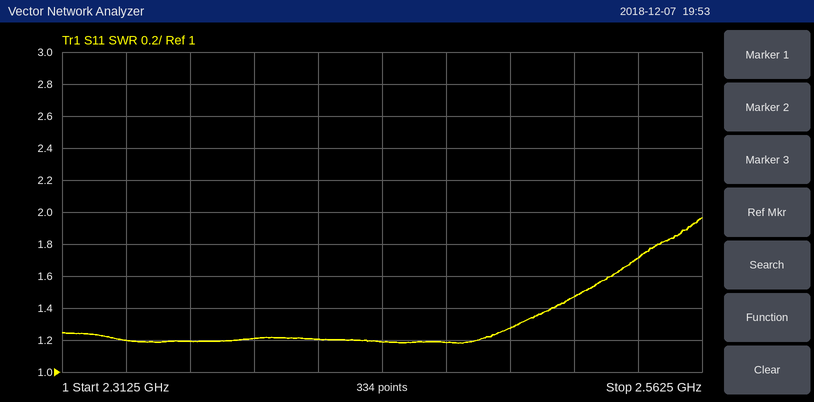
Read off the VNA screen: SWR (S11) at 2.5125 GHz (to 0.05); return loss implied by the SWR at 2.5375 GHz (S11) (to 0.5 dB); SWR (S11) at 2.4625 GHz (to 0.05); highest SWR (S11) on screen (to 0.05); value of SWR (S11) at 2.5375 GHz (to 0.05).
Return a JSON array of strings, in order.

["1.45", "11.5 dB", "1.20", "1.95", "1.70"]
